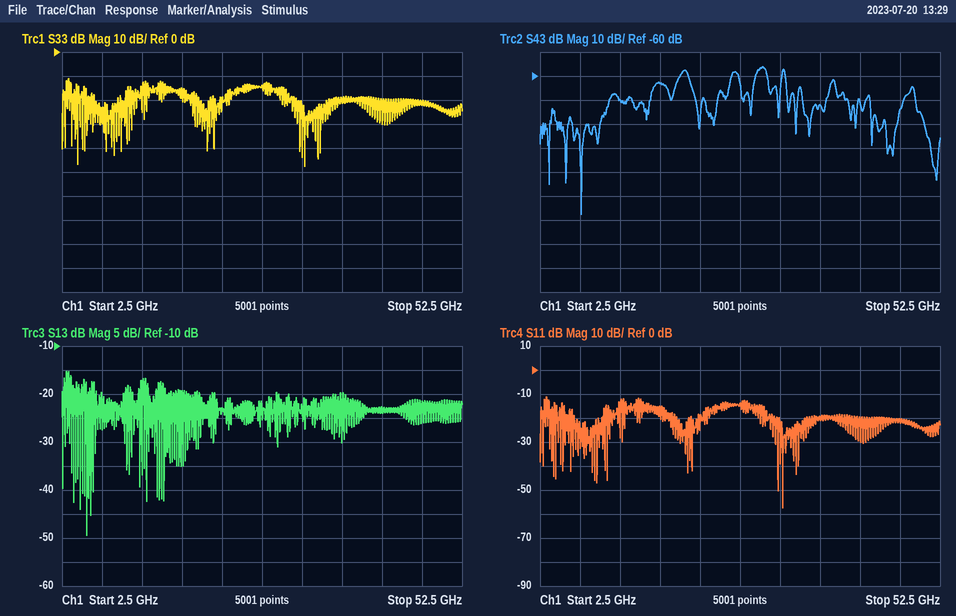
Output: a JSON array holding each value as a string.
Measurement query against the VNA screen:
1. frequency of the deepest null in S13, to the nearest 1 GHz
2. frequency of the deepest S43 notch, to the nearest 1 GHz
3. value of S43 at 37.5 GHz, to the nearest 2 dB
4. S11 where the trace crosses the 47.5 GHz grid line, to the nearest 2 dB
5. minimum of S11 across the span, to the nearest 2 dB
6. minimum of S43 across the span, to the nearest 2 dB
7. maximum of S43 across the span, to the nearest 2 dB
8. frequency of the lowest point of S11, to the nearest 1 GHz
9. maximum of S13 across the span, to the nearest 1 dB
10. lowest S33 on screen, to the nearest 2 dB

["6 GHz", "8 GHz", "-72 dB", "-22 dB", "-58 dB", "-118 dB", "-56 dB", "33 GHz", "-15 dB", "-48 dB"]
